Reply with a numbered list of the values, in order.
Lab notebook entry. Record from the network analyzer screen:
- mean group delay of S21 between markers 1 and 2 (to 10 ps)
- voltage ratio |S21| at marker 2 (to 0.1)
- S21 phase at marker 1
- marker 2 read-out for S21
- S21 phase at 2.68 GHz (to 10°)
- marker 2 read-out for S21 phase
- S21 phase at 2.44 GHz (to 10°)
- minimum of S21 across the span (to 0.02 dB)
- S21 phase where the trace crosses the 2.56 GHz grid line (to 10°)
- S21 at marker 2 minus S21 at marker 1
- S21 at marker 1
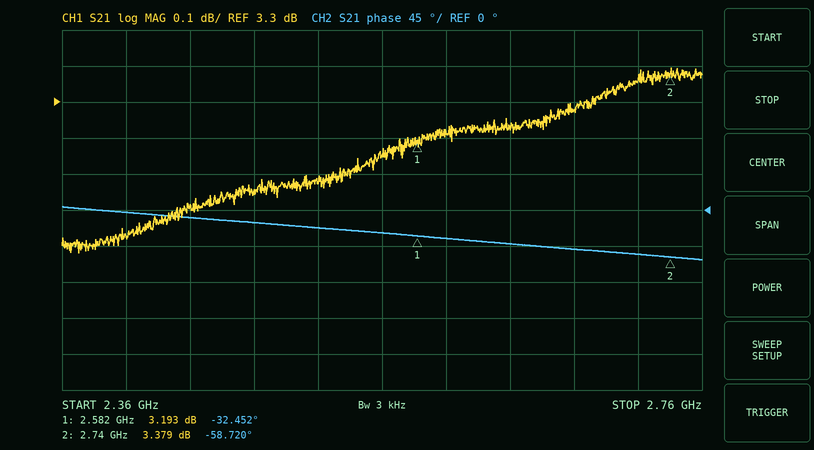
1. 460 ps
2. 1.5
3. -32.452°
4. 3.379 dB
5. -50°
6. -58.720°
7. -10°
8. 2.88 dB
9. -30°
10. 0.186 dB
11. 3.193 dB
